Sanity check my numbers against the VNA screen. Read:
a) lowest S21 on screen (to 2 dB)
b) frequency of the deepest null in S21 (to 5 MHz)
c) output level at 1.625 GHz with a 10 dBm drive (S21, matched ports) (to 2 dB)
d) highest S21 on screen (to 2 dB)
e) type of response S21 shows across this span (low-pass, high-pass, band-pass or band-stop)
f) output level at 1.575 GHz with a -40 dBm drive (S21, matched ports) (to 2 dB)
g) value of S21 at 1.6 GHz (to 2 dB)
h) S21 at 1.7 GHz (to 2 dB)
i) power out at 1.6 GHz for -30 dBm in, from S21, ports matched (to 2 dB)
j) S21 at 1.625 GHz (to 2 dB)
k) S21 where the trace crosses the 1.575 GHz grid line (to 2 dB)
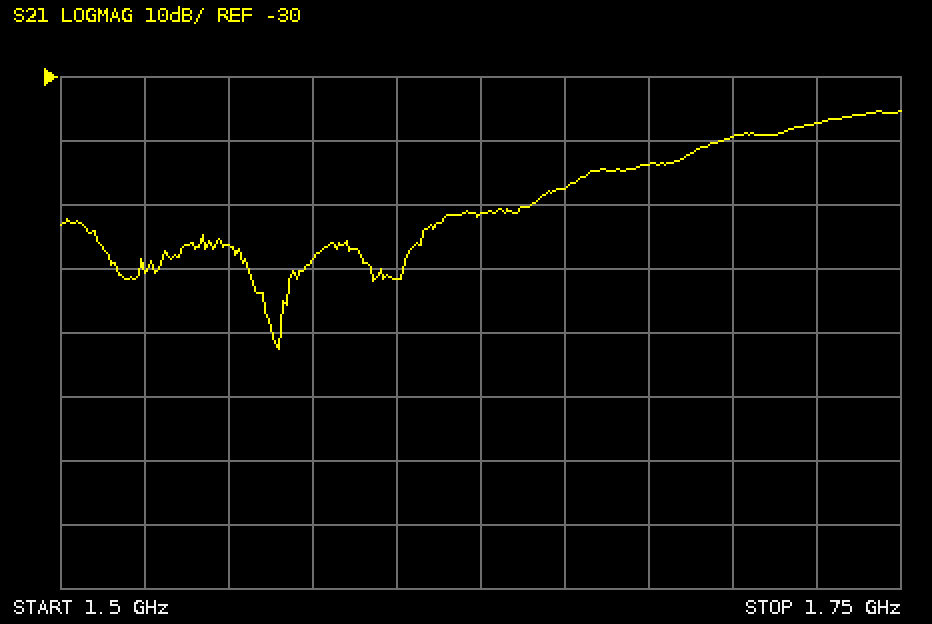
-72 dB
1.565 GHz
-42 dBm
-36 dB
high-pass
-98 dBm
-62 dB
-40 dB
-92 dBm
-52 dB
-58 dB
